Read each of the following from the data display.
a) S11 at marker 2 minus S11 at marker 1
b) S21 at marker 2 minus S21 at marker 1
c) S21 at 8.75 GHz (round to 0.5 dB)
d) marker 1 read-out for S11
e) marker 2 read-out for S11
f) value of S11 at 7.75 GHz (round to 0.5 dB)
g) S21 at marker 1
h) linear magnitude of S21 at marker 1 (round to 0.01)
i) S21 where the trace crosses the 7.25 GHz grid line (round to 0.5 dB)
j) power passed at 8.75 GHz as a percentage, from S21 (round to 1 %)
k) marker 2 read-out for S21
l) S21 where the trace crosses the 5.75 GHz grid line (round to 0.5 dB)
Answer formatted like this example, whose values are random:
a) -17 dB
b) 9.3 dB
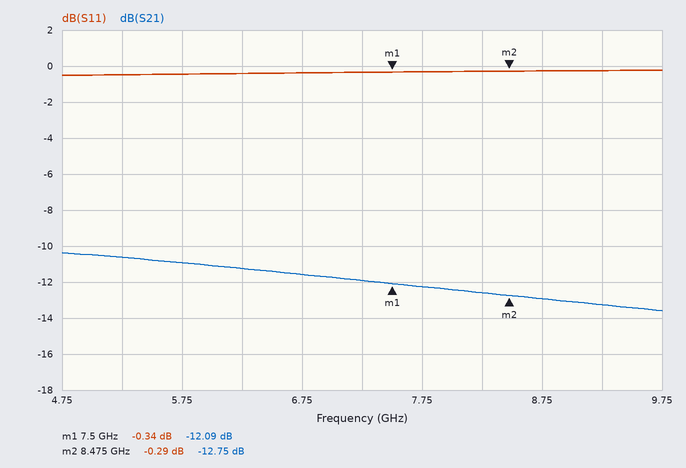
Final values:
a) 0.05 dB
b) -0.66 dB
c) -13.0 dB
d) -0.34 dB
e) -0.29 dB
f) -0.5 dB
g) -12.09 dB
h) 0.25
i) -12.0 dB
j) 5 %
k) -12.75 dB
l) -11.0 dB
